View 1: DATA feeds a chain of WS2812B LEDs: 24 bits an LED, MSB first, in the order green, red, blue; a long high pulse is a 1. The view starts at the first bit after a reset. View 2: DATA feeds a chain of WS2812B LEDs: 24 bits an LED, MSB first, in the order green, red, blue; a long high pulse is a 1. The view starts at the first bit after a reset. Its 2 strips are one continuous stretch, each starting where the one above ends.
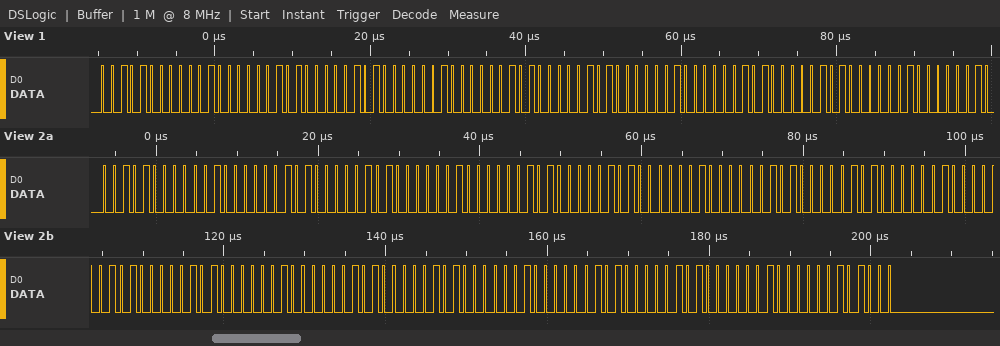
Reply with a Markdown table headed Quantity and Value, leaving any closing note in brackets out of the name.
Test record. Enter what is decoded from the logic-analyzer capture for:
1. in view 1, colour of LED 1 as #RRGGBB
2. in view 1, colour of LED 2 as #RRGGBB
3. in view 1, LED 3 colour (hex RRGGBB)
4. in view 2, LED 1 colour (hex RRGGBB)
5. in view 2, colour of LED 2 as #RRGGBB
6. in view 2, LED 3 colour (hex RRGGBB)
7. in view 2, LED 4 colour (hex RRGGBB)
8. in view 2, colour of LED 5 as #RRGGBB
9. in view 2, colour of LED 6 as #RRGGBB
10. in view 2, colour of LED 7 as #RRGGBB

| Quantity | Value |
|---|---|
| in view 1, colour of LED 1 as #RRGGBB | #102828 |
| in view 1, colour of LED 2 as #RRGGBB | #102828 |
| in view 1, LED 3 colour | #102828 |
| in view 2, LED 1 colour | #102828 |
| in view 2, colour of LED 2 as #RRGGBB | #102828 |
| in view 2, LED 3 colour | #102828 |
| in view 2, LED 4 colour | #102828 |
| in view 2, colour of LED 5 as #RRGGBB | #102828 |
| in view 2, colour of LED 6 as #RRGGBB | #102828 |
| in view 2, colour of LED 7 as #RRGGBB | #102828 |
